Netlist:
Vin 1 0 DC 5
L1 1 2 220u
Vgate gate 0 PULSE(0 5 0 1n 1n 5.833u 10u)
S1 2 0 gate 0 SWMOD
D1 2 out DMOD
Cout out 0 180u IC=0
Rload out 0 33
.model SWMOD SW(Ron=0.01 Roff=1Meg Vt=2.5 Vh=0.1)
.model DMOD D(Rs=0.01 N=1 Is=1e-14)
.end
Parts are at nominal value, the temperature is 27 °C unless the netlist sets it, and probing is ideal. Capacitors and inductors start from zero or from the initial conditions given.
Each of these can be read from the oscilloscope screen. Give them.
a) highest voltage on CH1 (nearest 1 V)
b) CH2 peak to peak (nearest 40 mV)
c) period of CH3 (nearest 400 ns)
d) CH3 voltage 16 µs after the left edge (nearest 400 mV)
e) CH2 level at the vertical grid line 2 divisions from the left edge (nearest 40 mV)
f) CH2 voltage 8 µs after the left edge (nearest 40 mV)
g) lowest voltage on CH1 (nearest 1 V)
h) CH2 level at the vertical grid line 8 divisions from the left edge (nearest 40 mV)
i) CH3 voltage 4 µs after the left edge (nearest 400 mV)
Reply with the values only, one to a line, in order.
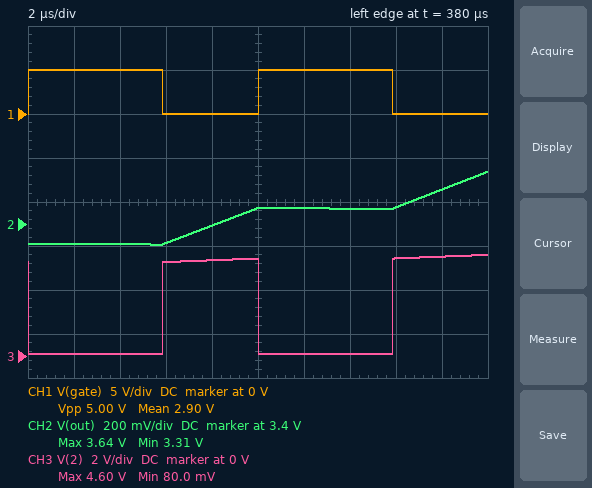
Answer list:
5 V
320 mV
10.0 µs
4.4 V
3.32 V
3.40 V
0 V
3.48 V
0 V
